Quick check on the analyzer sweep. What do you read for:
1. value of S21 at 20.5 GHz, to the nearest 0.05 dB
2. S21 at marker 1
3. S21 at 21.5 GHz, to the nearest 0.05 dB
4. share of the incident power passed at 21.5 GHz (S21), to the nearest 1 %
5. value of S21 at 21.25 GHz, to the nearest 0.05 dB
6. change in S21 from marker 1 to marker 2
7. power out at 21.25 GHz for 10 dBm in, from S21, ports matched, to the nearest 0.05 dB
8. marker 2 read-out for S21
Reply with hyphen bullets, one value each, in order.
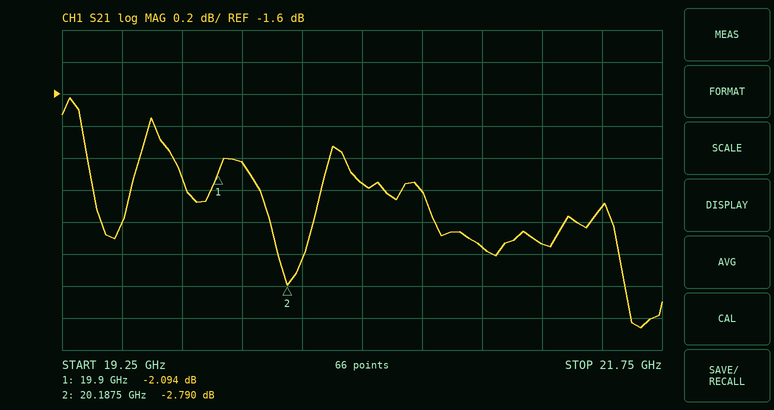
- -2.15 dB
- -2.094 dB
- -2.30 dB
- 59 %
- -2.55 dB
- -0.696 dB
- 7.45 dBm
- -2.790 dB
